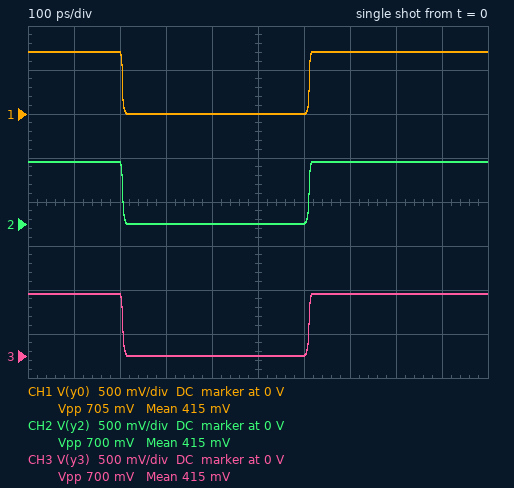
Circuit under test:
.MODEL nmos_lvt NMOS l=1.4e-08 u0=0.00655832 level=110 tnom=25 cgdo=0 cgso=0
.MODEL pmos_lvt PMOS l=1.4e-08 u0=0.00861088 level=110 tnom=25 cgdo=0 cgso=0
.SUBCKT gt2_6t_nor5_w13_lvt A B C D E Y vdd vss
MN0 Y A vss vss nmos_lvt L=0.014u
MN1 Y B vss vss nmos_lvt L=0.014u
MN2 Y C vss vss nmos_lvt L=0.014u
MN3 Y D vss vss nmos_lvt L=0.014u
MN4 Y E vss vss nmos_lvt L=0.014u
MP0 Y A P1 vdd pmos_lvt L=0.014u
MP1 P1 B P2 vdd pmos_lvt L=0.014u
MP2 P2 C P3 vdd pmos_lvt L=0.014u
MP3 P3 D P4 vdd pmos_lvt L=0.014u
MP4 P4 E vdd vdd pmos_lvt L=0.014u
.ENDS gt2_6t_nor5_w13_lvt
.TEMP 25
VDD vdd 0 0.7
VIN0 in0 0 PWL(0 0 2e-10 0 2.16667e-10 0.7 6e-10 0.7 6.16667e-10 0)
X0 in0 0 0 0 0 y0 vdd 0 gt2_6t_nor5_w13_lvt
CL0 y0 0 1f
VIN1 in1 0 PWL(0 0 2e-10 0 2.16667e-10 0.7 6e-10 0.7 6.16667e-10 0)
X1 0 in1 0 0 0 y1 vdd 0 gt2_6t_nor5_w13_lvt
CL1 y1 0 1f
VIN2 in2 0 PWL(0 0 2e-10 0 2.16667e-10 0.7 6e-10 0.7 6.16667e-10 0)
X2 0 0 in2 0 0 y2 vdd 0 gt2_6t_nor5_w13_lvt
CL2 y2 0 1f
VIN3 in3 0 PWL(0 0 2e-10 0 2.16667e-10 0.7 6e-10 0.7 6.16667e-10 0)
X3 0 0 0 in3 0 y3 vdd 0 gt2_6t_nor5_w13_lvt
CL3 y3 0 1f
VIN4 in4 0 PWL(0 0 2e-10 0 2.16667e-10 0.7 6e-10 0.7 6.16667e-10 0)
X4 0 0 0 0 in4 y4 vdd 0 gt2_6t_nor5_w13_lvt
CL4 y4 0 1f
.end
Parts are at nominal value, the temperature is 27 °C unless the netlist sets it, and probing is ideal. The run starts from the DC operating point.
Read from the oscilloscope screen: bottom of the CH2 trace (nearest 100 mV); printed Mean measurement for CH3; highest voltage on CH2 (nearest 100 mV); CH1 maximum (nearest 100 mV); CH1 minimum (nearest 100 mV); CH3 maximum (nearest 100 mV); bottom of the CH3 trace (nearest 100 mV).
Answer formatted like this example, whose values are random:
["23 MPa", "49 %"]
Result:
["0 V", "415 mV", "700 mV", "700 mV", "0 V", "700 mV", "0 V"]
